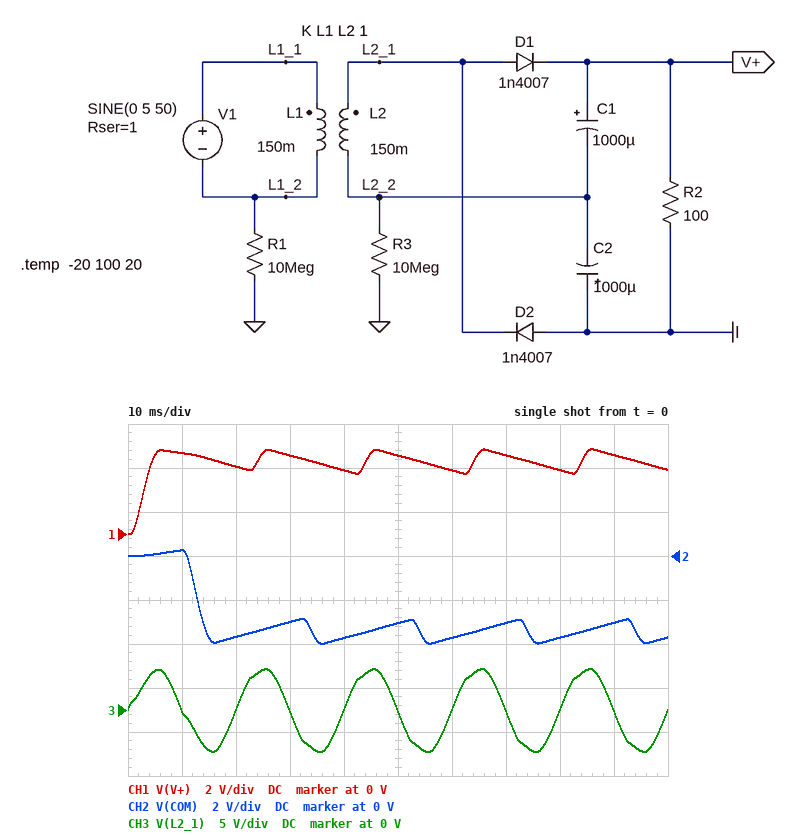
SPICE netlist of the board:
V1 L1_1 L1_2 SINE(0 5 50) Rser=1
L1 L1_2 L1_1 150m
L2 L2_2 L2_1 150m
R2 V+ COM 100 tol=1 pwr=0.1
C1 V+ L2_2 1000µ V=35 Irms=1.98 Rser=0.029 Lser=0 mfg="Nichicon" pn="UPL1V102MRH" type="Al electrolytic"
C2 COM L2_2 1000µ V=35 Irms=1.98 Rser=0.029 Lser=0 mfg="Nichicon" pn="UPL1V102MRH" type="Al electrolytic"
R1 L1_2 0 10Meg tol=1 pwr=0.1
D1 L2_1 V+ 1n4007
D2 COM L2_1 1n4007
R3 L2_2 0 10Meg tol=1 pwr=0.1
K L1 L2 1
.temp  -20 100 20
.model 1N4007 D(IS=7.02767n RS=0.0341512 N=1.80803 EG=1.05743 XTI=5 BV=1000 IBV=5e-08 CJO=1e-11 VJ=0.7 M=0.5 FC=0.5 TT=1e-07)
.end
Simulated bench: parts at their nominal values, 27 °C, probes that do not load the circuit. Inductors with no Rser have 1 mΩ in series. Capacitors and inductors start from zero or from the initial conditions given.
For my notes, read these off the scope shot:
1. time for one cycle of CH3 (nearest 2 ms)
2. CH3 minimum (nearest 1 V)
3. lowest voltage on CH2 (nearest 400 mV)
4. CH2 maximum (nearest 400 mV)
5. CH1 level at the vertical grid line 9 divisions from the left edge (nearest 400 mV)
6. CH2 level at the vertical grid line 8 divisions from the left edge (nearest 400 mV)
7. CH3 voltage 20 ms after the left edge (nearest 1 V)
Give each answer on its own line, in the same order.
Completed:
20 ms
-5 V
-4.0 V
400 mV
3.6 V
-3.6 V
0 V
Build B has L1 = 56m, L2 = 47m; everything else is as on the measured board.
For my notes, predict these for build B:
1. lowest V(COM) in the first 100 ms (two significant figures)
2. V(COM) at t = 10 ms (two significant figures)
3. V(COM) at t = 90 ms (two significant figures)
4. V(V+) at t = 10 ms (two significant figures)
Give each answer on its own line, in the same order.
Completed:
-3.7 V
230 mV
-2.8 V
3.2 V
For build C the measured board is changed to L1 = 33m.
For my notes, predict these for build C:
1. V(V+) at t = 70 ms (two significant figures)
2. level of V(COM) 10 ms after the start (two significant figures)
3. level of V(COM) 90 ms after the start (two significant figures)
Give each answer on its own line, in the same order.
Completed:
6.6 V
330 mV
-5.8 V
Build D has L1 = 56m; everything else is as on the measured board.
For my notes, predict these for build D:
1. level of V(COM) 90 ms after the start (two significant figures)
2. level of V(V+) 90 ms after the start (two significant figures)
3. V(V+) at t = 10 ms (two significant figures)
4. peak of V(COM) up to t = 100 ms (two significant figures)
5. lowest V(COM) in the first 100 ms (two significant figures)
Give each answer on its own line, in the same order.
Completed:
-4.8 V
5.6 V
5.2 V
340 mV
-6.3 V
